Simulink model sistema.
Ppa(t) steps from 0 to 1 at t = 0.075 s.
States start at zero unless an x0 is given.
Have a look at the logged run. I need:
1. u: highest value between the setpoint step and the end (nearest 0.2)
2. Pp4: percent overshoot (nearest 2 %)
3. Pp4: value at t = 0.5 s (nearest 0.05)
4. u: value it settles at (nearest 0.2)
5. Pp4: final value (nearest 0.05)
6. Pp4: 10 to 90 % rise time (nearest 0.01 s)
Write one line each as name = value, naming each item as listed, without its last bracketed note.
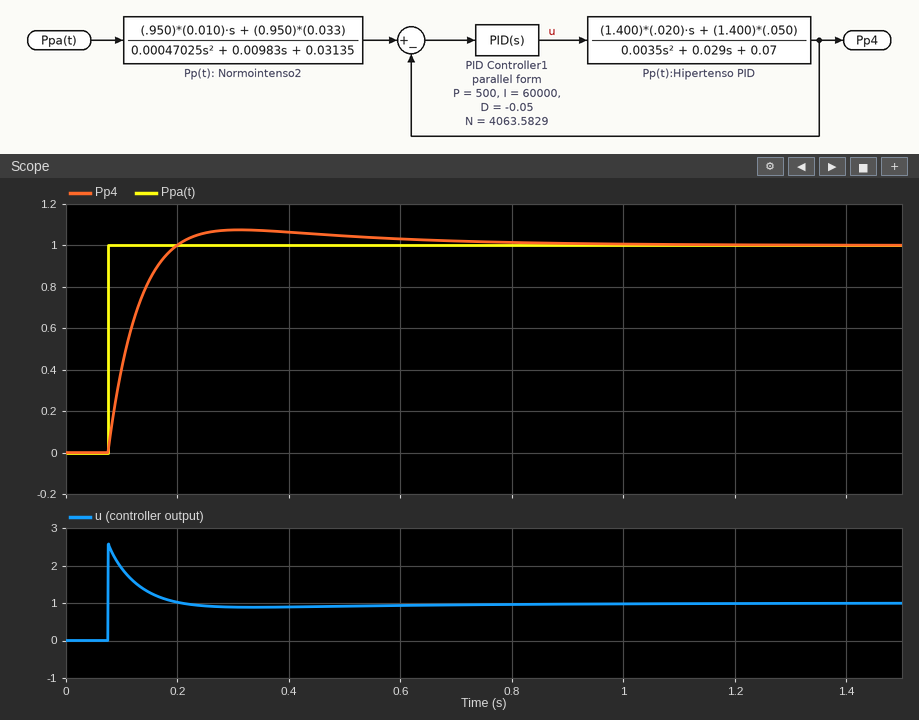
u: highest value between the setpoint step and the end = 2.6
Pp4: percent overshoot = 8 %
Pp4: value at t = 0.5 s = 1.05
u: value it settles at = 1.0
Pp4: final value = 1.00
Pp4: 10 to 90 % rise time = 0.08 s
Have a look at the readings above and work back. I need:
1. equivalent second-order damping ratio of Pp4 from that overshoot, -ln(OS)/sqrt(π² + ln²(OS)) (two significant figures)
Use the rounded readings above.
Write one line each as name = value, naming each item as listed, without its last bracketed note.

equivalent second-order damping ratio of Pp4 from that overshoot, -ln(OS)/sqrt(π² + ln²(OS)) = 0.63
